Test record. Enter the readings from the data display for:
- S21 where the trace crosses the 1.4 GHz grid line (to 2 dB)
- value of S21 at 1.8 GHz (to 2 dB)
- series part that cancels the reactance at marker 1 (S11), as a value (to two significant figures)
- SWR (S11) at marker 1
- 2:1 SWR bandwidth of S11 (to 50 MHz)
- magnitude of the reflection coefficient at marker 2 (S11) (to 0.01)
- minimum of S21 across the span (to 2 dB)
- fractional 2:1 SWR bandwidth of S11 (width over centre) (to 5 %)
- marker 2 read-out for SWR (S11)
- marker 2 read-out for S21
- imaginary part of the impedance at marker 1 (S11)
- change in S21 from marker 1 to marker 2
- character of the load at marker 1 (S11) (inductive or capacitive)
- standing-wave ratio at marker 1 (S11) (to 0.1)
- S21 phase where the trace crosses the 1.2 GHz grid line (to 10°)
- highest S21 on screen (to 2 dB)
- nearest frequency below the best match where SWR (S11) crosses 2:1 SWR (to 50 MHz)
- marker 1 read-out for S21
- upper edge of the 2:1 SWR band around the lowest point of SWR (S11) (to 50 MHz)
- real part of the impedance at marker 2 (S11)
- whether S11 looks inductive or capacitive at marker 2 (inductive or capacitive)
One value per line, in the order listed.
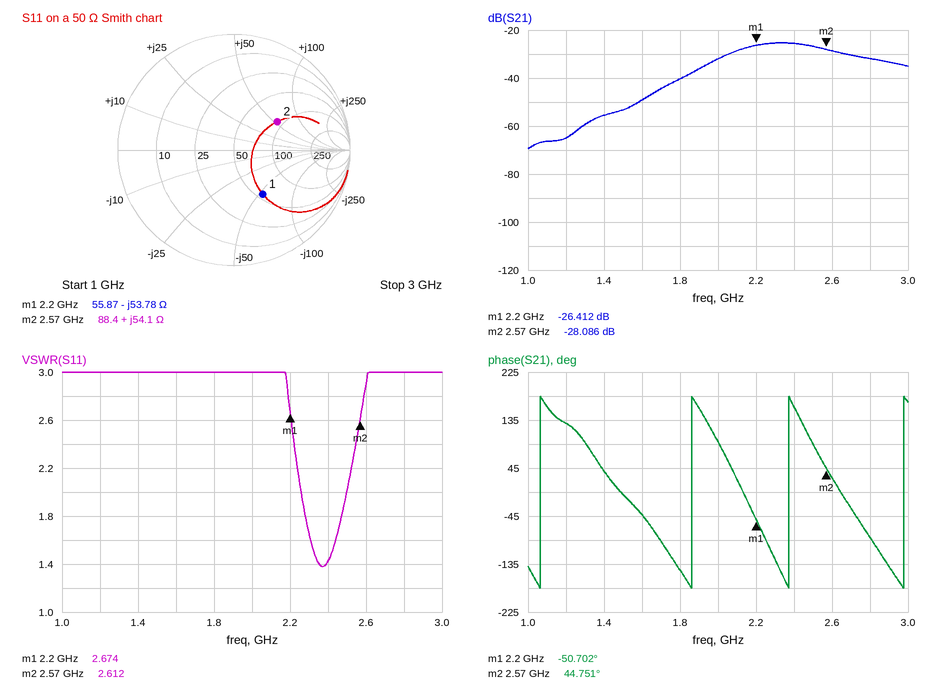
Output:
-56 dB
-40 dB
3.9 nH
2.674
250 MHz
0.45
-70 dB
10 %
2.612
-28.086 dB
-53.78 Ω
-1.674 dB
capacitive
2.7
130°
-26 dB
2.25 GHz
-26.412 dB
2.50 GHz
88.4 Ω
inductive
